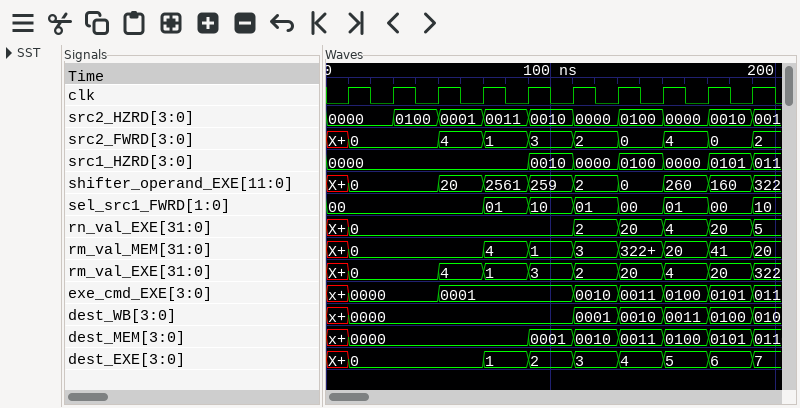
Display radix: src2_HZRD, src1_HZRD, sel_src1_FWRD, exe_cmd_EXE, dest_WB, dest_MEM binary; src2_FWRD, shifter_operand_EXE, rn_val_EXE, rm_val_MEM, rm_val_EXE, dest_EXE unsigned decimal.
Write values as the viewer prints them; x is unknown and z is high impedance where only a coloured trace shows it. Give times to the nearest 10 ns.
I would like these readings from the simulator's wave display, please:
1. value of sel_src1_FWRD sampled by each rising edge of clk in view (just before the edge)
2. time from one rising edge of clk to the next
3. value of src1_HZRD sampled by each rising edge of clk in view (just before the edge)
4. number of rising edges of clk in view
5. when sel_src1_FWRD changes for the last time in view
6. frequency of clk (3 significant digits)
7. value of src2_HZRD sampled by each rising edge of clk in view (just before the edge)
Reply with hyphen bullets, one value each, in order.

- 00, 00, 00, 00, 01, 10, 01, 00, 01, 00
- 20 ns
- 0000, 0000, 0000, 0000, 0000, 0010, 0000, 0100, 0000, 0101
- 10
- 190 ns
- 50.0 MHz
- 0000, 0000, 0100, 0001, 0011, 0010, 0000, 0100, 0000, 0010
